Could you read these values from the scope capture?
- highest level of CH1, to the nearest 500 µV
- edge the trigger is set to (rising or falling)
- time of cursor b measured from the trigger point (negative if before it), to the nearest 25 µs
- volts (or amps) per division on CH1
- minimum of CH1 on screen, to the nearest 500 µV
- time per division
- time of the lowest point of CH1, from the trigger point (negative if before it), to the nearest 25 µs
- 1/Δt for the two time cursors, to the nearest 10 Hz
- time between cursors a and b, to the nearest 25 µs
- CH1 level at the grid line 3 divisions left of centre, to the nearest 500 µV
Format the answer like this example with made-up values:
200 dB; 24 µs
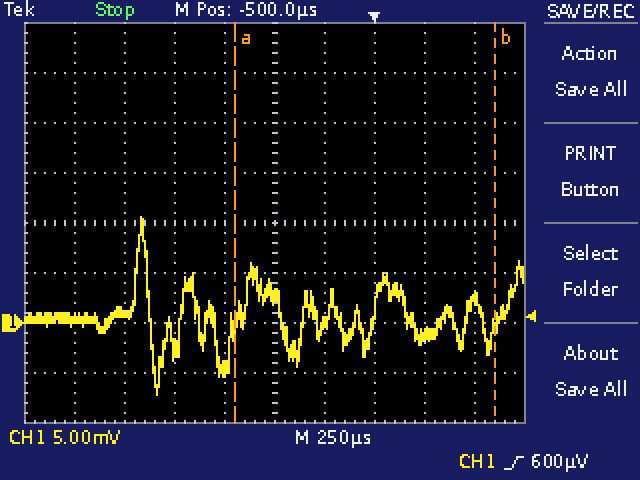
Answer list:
10.5 mV; rising; +600 µs; 5 mV; -7.0 mV; 250 µs; -1.075 ms; 770 Hz; 1.300 ms; 1.0 mV
